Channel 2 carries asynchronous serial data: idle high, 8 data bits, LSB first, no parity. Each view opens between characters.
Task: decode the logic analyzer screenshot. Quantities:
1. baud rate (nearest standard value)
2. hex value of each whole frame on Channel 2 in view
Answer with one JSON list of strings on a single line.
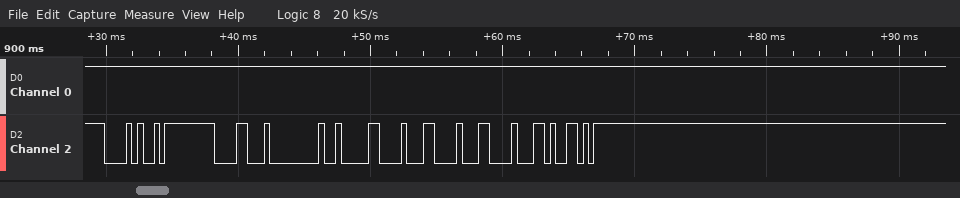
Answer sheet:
["2400 baud", "28, FF, 18, 00, 82, 88, 88, 88, 59"]
